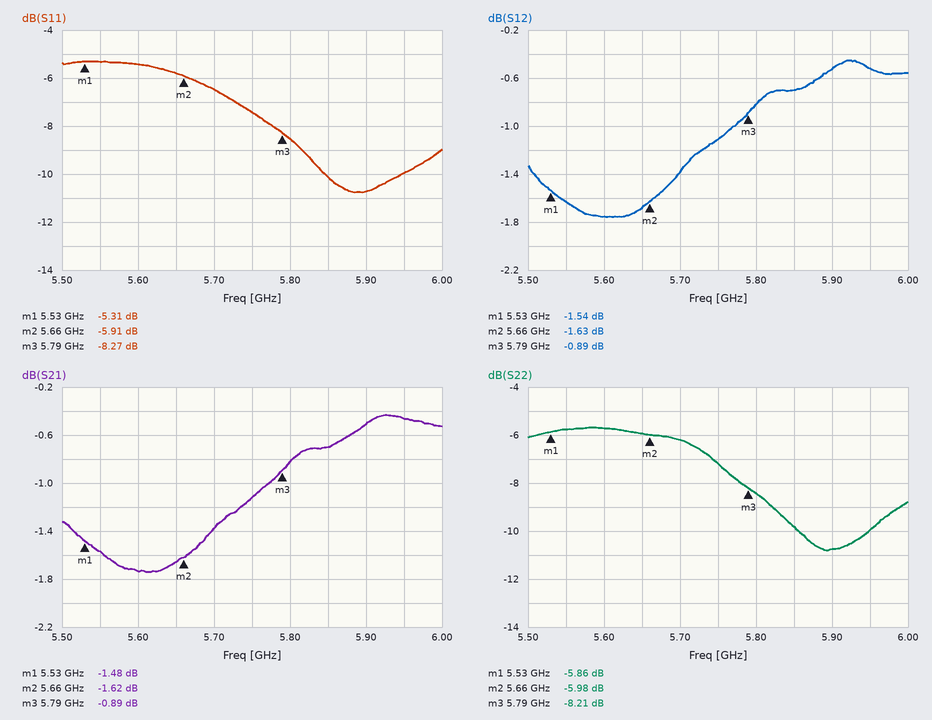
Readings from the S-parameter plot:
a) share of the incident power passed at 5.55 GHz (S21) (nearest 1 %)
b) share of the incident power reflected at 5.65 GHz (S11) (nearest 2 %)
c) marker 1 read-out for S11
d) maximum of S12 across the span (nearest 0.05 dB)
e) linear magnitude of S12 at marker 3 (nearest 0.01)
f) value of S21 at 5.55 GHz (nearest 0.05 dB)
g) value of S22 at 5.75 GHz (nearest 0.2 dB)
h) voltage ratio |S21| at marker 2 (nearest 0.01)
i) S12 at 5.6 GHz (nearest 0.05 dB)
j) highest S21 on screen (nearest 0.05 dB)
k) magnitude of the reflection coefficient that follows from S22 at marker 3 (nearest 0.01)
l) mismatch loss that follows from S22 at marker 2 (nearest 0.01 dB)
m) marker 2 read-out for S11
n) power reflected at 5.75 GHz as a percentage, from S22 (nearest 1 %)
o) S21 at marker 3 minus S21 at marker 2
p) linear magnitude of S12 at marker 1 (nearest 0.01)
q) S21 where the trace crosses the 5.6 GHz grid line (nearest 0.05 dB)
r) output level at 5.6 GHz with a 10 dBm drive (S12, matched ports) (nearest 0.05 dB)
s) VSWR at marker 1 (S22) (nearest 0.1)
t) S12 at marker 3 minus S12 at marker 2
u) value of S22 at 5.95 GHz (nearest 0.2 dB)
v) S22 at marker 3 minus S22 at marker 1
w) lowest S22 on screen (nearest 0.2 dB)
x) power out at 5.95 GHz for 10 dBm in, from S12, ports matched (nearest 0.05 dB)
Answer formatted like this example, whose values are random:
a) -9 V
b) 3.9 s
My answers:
a) 70 %
b) 26 %
c) -5.31 dB
d) -0.45 dB
e) 0.90
f) -1.55 dB
g) -7.2 dB
h) 0.83
i) -1.75 dB
j) -0.45 dB
k) 0.39
l) 1.26 dB
m) -5.91 dB
n) 19 %
o) 0.73 dB
p) 0.84
q) -1.75 dB
r) 8.25 dBm
s) 3.1
t) 0.74 dB
u) -10.0 dB
v) -2.35 dB
w) -10.8 dB
x) 9.50 dBm
